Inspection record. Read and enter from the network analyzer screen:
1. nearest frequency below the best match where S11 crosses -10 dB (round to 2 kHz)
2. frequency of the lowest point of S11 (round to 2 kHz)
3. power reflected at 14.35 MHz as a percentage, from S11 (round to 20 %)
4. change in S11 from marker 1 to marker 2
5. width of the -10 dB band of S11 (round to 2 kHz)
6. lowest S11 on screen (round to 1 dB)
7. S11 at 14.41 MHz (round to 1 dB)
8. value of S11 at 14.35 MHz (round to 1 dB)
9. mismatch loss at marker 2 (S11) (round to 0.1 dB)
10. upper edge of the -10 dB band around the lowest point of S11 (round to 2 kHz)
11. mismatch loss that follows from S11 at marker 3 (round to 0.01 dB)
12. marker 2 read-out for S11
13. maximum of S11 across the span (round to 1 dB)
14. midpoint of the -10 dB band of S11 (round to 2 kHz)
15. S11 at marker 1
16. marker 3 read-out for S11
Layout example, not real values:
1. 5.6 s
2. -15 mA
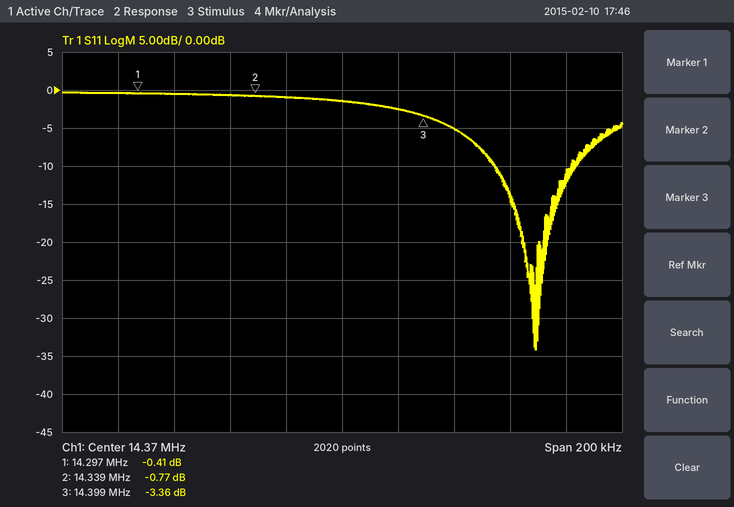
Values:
1. 14.424 MHz
2. 14.440 MHz
3. 80 %
4. -0.36 dB
5. 28 kHz
6. -34 dB
7. -5 dB
8. -1 dB
9. 7.9 dB
10. 14.452 MHz
11. 2.69 dB
12. -0.77 dB
13. 0 dB
14. 14.438 MHz
15. -0.41 dB
16. -3.36 dB
